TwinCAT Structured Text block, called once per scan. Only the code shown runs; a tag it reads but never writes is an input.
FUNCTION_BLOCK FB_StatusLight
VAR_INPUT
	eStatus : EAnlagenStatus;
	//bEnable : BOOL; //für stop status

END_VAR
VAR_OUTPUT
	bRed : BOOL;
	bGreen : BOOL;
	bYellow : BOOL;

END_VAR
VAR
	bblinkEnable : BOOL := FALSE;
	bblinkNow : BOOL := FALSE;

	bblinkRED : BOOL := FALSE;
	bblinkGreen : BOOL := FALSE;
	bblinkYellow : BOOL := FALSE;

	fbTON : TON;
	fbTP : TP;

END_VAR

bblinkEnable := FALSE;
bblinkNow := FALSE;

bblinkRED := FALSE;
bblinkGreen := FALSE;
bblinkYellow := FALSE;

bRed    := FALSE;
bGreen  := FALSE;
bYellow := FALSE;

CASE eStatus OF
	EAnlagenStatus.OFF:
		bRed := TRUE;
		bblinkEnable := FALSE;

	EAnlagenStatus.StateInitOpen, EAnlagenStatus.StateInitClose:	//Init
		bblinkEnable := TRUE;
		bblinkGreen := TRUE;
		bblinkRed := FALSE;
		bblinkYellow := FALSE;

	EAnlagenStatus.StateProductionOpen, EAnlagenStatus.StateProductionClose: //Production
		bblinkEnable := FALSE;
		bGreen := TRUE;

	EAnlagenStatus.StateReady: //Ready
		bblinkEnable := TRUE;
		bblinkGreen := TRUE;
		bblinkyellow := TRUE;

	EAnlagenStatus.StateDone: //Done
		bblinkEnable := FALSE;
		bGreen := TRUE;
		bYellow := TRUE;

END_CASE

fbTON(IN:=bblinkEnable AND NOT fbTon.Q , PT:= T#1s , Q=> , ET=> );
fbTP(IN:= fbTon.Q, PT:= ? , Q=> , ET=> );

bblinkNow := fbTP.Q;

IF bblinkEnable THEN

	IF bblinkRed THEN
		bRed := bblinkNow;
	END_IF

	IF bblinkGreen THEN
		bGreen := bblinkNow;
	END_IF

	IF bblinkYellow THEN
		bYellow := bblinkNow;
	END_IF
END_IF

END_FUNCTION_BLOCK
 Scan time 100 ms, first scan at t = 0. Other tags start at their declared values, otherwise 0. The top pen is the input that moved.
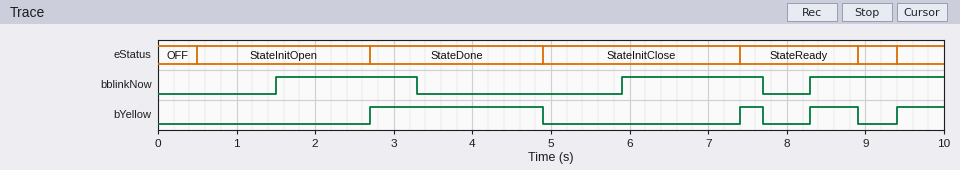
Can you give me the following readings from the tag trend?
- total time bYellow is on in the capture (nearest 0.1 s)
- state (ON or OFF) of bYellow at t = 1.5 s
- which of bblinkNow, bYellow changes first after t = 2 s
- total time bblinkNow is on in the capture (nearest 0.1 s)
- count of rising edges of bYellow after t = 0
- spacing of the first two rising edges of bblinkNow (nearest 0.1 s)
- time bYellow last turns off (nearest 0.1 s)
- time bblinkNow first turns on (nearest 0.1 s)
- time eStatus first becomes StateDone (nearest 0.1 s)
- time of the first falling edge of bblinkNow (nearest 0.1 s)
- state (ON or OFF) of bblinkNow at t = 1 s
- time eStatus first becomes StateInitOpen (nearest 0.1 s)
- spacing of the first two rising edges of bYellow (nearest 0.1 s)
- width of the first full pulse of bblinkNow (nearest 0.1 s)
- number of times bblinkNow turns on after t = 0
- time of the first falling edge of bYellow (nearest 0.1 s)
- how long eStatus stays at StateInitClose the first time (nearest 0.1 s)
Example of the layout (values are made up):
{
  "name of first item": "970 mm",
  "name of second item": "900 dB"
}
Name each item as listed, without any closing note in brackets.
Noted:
{
  "total time bYellow is on in the capture": "3.7 s",
  "state (ON or OFF) of bYellow at t = 1.5 s": "OFF",
  "which of bblinkNow, bYellow changes first after t = 2 s": "bYellow",
  "total time bblinkNow is on in the capture": "5.3 s",
  "count of rising edges of bYellow after t = 0": "4",
  "spacing of the first two rising edges of bblinkNow": "4.4 s",
  "time bYellow last turns off": "8.9 s",
  "time bblinkNow first turns on": "1.5 s",
  "time eStatus first becomes StateDone": "2.7 s",
  "time of the first falling edge of bblinkNow": "3.3 s",
  "state (ON or OFF) of bblinkNow at t = 1 s": "OFF",
  "time eStatus first becomes StateInitOpen": "0.5 s",
  "spacing of the first two rising edges of bYellow": "4.7 s",
  "width of the first full pulse of bblinkNow": "1.8 s",
  "number of times bblinkNow turns on after t = 0": "3",
  "time of the first falling edge of bYellow": "4.9 s",
  "how long eStatus stays at StateInitClose the first time": "2.5 s"
}
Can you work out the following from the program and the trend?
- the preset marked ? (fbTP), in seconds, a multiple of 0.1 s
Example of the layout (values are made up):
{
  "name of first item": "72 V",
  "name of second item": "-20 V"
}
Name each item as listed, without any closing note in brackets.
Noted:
{
  "the preset marked ? (fbTP), in seconds, a multiple of 0.1 s": "1.8 s"
}
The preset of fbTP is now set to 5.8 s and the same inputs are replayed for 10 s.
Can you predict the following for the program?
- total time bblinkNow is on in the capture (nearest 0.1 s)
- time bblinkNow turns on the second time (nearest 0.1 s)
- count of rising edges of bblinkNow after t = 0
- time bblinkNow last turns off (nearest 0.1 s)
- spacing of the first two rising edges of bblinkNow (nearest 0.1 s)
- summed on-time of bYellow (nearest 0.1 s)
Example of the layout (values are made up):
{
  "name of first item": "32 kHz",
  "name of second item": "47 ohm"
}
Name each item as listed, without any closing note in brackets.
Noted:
{
  "total time bblinkNow is on in the capture": "7.5 s",
  "time bblinkNow turns on the second time": "8.3 s",
  "count of rising edges of bblinkNow after t = 0": "2",
  "time bblinkNow last turns off": "7.3 s",
  "spacing of the first two rising edges of bblinkNow": "6.8 s",
  "summed on-time of bYellow": "3.4 s"
}
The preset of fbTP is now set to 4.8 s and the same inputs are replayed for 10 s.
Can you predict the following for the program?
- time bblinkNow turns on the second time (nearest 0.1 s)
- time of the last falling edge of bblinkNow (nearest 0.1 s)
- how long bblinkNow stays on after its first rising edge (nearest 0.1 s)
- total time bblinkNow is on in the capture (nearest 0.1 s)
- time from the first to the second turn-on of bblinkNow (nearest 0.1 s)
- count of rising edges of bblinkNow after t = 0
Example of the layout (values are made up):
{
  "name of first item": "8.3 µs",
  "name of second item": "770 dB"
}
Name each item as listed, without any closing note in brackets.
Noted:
{
  "time bblinkNow turns on the second time": "7.1 s",
  "time of the last falling edge of bblinkNow": "6.3 s",
  "how long bblinkNow stays on after its first rising edge": "4.8 s",
  "total time bblinkNow is on in the capture": "7.7 s",
  "time from the first to the second turn-on of bblinkNow": "5.6 s",
  "count of rising edges of bblinkNow after t = 0": "2"
}
